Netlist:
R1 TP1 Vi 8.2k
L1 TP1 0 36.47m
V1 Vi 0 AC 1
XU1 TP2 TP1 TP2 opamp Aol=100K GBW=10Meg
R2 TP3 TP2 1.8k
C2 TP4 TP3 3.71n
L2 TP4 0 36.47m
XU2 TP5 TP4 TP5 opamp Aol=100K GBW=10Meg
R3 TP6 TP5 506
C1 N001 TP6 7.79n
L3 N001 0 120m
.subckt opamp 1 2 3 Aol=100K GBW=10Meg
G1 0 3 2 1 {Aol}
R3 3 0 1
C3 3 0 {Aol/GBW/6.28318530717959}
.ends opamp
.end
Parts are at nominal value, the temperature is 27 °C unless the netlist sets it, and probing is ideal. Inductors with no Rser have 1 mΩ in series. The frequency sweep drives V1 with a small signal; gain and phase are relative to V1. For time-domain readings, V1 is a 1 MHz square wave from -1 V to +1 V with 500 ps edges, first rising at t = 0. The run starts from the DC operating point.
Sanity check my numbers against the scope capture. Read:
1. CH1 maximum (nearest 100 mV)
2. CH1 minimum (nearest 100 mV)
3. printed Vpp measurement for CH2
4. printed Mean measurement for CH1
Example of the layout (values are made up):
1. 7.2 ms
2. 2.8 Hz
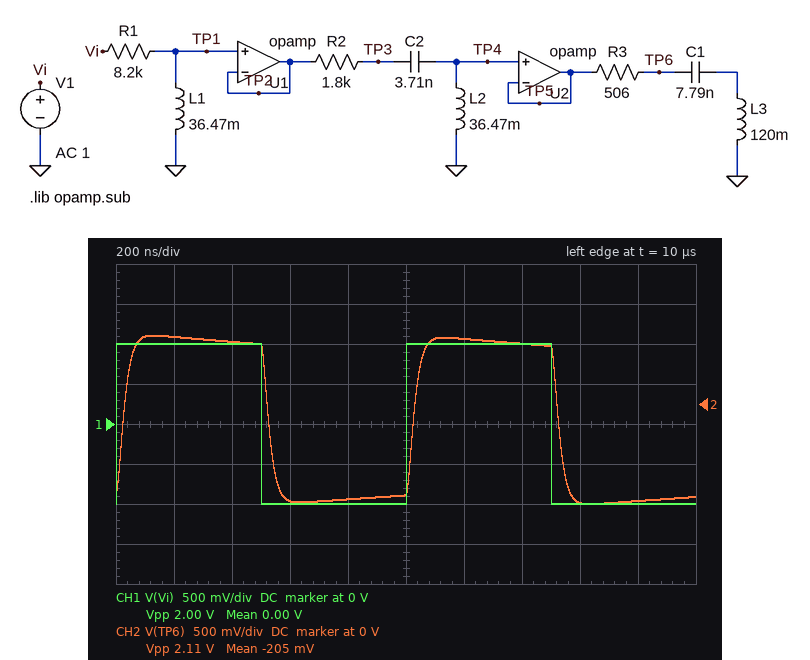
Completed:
1. 1.0 V
2. -1.0 V
3. 2.11 V
4. 0.00 V
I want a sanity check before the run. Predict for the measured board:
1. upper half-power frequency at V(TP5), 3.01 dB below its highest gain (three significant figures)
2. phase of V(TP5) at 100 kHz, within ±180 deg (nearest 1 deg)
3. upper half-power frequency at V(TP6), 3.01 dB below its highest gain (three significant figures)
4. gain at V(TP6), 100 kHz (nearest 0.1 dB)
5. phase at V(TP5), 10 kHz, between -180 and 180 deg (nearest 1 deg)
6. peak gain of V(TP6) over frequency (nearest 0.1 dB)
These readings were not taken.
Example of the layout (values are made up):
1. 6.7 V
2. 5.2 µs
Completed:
1. 6.48 MHz
2. 23 deg
3. 6.48 MHz
4. -0.4 dB
5. -148 deg
6. 0 dB
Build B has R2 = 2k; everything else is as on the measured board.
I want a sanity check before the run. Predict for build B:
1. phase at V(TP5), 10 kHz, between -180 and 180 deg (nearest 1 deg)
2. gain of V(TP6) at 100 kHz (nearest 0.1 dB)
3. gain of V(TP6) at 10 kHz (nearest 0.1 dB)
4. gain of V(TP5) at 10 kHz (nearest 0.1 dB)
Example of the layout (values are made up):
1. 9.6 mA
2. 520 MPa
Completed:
1. -151 deg
2. -0.4 dB
3. -13.3 dB
4. -13.2 dB
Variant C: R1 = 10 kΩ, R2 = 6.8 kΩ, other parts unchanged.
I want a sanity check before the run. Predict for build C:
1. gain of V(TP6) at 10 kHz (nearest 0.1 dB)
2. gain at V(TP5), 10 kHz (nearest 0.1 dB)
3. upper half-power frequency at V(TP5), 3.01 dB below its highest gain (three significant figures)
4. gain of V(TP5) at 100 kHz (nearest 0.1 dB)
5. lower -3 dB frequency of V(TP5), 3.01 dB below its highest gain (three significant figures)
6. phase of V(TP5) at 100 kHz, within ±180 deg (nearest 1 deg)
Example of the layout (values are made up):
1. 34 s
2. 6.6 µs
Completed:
1. -22.9 dB
2. -22.8 dB
3. 6.51 MHz
4. -1.0 dB
5. 52.1 kHz
6. 39 deg
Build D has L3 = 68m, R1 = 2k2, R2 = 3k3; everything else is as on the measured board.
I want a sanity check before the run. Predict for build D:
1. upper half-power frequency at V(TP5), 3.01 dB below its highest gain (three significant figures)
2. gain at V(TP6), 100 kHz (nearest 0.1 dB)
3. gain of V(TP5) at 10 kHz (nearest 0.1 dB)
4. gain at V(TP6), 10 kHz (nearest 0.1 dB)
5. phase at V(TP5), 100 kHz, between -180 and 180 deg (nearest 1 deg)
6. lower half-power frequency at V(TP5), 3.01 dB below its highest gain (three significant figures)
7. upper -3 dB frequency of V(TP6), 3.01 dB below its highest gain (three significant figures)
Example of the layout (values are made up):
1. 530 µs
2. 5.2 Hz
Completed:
1. 6.11 MHz
2. 0 dB
3. -7.4 dB
4. -7.6 dB
5. 13 deg
6. 13.1 kHz
7. 6.12 MHz
